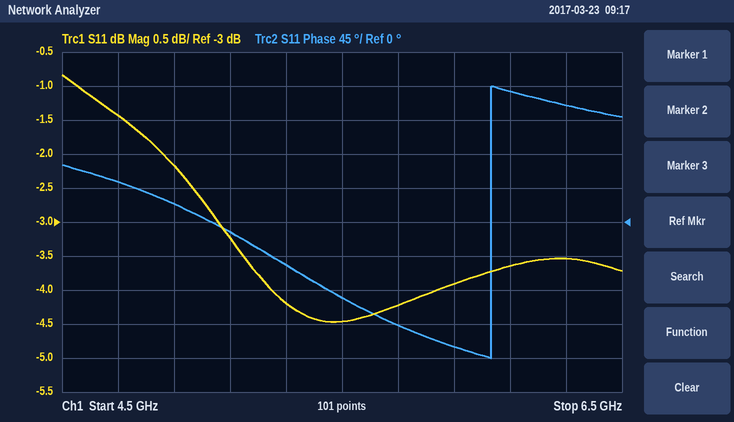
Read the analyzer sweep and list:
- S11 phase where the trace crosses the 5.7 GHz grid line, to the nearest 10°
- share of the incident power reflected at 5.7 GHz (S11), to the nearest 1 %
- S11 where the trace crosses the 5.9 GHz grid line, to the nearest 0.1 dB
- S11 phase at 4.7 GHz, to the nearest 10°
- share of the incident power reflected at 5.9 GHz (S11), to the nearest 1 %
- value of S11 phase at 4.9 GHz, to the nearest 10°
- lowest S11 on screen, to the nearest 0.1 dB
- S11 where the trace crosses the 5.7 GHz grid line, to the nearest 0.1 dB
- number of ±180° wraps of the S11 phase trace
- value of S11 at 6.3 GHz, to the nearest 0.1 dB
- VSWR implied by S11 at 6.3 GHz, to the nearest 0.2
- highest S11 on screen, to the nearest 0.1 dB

-140°
38 %
-3.9 dB
50°
41 %
20°
-4.5 dB
-4.2 dB
1
-3.5 dB
5.0
-0.8 dB
